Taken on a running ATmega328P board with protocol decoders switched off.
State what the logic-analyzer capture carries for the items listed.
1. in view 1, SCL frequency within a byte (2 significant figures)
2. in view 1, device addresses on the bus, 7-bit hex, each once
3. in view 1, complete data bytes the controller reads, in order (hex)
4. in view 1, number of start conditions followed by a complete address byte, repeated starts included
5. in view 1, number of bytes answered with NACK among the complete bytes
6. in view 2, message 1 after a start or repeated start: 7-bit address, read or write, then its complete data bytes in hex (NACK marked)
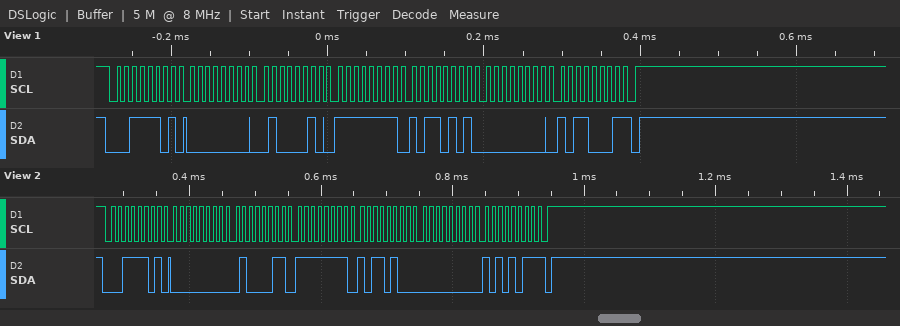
100 kHz
0x1E
00 42 FF B5 00 B1
1
1
0x1E read: 00 43 FF B4 00 AB NACK
